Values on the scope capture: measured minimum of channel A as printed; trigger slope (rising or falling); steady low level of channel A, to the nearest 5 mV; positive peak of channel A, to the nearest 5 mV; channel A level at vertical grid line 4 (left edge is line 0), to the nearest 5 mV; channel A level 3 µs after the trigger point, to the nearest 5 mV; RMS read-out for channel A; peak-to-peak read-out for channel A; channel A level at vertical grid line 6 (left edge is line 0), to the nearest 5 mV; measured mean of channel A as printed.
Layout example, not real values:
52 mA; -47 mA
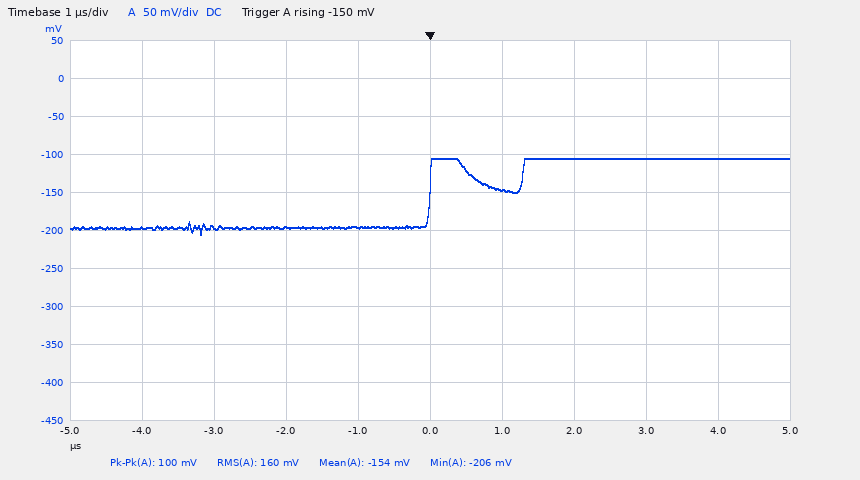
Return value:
-206 mV; rising; -195 mV; -105 mV; -195 mV; -105 mV; 160 mV; 100 mV; -145 mV; -154 mV
